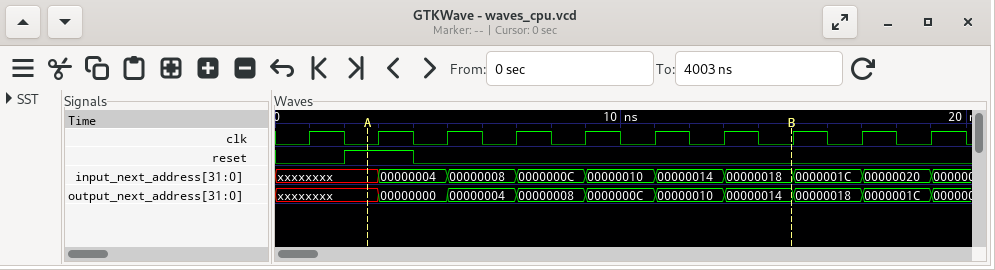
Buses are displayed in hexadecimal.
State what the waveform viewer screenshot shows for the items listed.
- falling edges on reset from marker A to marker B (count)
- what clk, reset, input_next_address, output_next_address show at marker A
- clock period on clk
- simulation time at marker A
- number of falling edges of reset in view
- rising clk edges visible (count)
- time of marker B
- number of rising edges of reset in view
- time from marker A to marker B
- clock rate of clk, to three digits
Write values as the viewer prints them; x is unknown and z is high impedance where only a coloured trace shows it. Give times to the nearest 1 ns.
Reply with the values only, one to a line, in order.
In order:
1
clk=0, reset=1, input_next_address=xxxxxxxx, output_next_address=xxxxxxxx
2 ns
3 ns
1
10
15 ns
1
12 ns
500 MHz
